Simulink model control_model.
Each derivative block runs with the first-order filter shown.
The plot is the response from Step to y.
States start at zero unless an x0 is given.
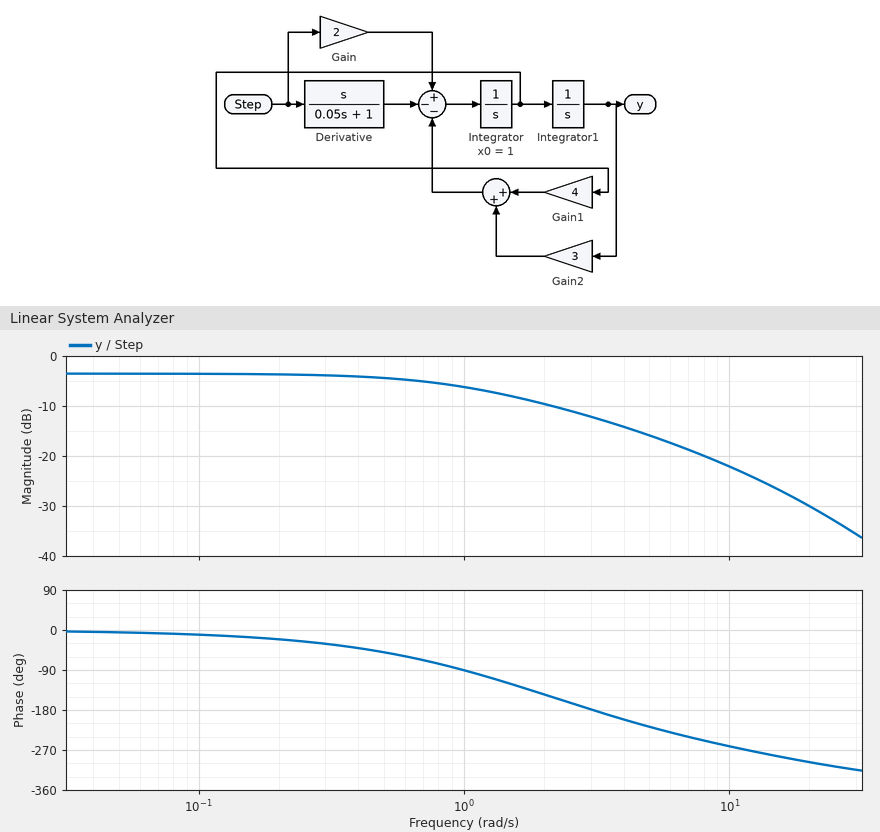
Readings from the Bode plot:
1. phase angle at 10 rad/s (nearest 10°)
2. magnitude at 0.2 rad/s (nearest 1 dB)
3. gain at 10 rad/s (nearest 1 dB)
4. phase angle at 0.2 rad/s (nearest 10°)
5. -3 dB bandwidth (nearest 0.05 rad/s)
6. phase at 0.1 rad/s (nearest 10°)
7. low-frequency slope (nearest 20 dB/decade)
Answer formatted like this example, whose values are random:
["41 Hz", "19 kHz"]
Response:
["-260°", "-4 dB", "-22 dB", "-20°", "1.10 rad/s", "-10°", "0 dB/decade"]
